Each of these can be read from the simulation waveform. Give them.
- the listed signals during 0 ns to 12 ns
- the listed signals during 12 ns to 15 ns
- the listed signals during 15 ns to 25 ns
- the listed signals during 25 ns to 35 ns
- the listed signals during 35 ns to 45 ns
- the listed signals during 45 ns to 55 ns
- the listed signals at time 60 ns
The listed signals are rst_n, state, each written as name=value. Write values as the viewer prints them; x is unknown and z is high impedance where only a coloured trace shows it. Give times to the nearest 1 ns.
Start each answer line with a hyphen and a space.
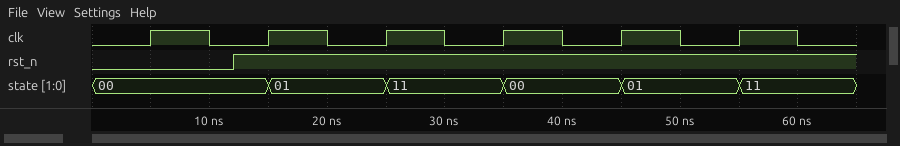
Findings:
- rst_n=0, state=00
- rst_n=1, state=00
- rst_n=1, state=01
- rst_n=1, state=11
- rst_n=1, state=00
- rst_n=1, state=01
- rst_n=1, state=11
